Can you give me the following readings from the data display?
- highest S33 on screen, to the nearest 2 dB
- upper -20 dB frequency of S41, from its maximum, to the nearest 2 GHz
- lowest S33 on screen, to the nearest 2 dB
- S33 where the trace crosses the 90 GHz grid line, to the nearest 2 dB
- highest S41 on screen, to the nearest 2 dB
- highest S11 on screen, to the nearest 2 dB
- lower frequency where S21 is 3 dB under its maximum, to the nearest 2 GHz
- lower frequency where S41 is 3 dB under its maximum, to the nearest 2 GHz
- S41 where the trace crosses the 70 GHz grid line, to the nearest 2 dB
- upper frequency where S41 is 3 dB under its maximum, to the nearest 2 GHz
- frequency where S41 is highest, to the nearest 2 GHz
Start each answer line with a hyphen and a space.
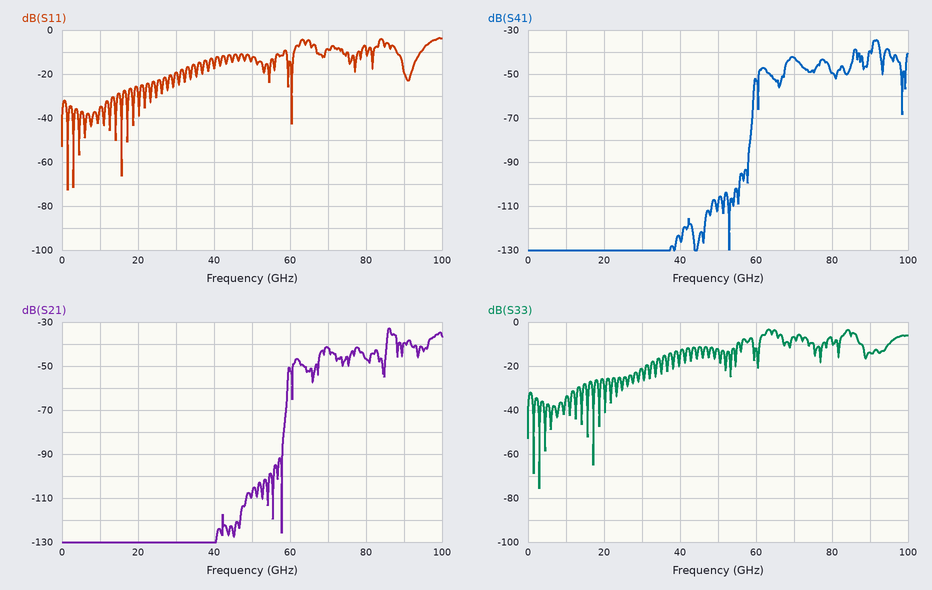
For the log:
- -4 dB
- 98 GHz
- -76 dB
- -14 dB
- -34 dB
- -4 dB
- 86 GHz
- 90 GHz
- -42 dB
- 92 GHz
- 92 GHz
